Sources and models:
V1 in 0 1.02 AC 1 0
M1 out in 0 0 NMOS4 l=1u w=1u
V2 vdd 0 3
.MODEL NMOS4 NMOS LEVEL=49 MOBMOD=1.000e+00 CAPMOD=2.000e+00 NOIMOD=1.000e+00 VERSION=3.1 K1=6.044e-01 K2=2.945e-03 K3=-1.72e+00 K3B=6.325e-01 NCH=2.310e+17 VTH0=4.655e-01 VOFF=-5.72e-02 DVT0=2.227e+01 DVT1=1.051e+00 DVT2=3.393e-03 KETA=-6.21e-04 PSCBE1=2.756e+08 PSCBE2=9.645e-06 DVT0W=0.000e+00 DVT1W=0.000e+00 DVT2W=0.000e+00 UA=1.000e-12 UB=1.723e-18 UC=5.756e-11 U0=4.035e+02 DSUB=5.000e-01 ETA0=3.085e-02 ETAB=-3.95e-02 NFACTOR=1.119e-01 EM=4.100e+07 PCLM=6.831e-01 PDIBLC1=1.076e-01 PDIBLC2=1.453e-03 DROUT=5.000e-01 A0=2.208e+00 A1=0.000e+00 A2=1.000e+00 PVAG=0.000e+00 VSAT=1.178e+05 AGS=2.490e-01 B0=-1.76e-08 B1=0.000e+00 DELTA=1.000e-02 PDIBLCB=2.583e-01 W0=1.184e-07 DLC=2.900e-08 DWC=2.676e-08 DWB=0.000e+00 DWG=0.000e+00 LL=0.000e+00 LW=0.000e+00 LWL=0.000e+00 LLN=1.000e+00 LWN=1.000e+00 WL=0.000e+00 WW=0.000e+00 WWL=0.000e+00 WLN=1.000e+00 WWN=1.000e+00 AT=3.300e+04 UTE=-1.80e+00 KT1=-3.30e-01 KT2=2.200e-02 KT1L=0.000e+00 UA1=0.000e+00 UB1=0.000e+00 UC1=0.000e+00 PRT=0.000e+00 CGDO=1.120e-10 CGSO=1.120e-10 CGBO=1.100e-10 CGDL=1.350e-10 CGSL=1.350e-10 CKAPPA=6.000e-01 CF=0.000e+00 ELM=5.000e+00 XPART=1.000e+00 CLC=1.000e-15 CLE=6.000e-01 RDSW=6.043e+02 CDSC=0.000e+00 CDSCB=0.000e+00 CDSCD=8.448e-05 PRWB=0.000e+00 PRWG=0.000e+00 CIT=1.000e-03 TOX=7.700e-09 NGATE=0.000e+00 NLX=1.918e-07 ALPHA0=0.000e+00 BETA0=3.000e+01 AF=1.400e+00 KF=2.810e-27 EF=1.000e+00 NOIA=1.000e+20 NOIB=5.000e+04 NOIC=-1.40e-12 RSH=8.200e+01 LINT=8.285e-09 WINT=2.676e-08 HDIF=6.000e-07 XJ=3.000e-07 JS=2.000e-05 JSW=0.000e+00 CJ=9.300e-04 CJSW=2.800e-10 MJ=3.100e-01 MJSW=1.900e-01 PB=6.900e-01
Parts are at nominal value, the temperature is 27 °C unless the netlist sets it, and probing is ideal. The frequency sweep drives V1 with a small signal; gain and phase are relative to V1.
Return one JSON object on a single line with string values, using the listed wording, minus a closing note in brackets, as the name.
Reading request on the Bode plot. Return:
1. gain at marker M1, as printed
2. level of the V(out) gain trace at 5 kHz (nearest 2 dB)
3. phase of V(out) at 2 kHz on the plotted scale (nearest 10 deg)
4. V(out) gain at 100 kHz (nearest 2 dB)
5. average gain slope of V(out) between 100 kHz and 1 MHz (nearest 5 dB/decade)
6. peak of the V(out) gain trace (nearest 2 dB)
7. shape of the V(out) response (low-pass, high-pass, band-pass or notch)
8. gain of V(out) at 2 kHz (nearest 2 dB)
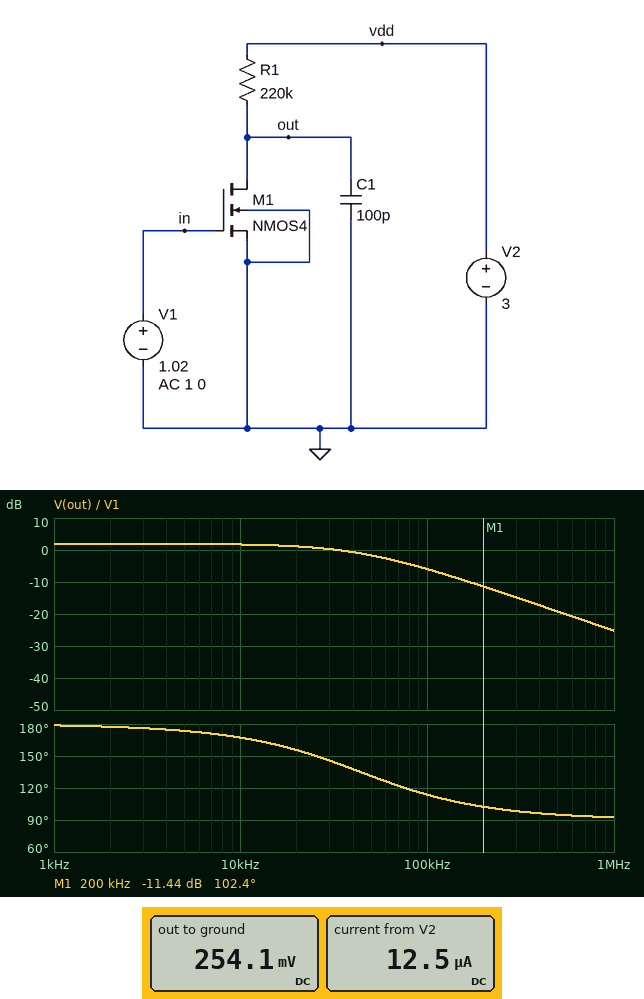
{"gain at marker M1, as printed": "-11.44 dB", "level of the V(out) gain trace at 5 kHz": "2 dB", "phase of V(out) at 2 kHz on the plotted scale": "180 deg", "V(out) gain at 100 kHz": "-6 dB", "average gain slope of V(out) between 100 kHz and 1 MHz": "-20 dB/decade", "peak of the V(out) gain trace": "2 dB", "shape of the V(out) response": "low-pass", "gain of V(out) at 2 kHz": "2 dB"}
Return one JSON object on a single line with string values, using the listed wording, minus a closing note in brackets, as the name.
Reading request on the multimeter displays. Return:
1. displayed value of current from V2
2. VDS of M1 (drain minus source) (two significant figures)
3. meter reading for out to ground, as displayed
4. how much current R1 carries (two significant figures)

{"displayed value of current from V2": "12.5 µA", "VDS of M1 (drain minus source)": "250 mV", "meter reading for out to ground, as displayed": "254.1 mV", "how much current R1 carries": "12 µA"}
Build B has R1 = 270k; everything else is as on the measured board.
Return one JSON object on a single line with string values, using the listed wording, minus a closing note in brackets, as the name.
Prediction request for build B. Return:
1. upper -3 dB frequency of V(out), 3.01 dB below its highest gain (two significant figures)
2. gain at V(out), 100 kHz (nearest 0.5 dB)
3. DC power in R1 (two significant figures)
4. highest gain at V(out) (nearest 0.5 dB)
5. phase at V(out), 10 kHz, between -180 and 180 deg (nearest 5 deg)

{"upper -3 dB frequency of V(out), 3.01 dB below its highest gain": "64 kHz", "gain at V(out), 100 kHz": "-9.5 dB", "DC power in R1": "29 µW", "highest gain at V(out)": "-4.0 dB", "phase at V(out), 10 kHz, between -180 and 180 deg": "170 deg"}
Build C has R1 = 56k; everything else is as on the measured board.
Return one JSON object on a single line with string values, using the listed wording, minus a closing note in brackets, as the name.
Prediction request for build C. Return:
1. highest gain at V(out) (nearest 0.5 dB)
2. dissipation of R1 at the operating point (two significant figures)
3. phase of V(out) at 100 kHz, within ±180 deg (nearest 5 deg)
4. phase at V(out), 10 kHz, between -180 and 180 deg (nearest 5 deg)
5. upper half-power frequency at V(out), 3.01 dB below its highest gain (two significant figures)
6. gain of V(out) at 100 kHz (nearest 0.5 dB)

{"highest gain at V(out)": "9.5 dB", "dissipation of R1 at the operating point": "13 µW", "phase of V(out) at 100 kHz, within ±180 deg": "105 deg", "phase at V(out), 10 kHz, between -180 and 180 deg": "160 deg", "upper half-power frequency at V(out), 3.01 dB below its highest gain": "29 kHz", "gain of V(out) at 100 kHz": "-2.0 dB"}
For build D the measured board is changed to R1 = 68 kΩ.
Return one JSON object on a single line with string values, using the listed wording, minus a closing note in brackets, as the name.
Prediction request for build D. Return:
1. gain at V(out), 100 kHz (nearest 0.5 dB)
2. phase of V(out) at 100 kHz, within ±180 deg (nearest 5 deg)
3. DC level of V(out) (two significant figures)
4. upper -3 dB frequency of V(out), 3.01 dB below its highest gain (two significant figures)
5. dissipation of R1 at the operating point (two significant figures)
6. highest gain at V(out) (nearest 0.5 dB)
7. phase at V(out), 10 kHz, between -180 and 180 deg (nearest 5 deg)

{"gain at V(out), 100 kHz": "-1.5 dB", "phase of V(out) at 100 kHz, within ±180 deg": "105 deg", "DC level of V(out)": "2.0 V", "upper -3 dB frequency of V(out), 3.01 dB below its highest gain": "24 kHz", "dissipation of R1 at the operating point": "15 µW", "highest gain at V(out)": "11.0 dB", "phase at V(out), 10 kHz, between -180 and 180 deg": "155 deg"}
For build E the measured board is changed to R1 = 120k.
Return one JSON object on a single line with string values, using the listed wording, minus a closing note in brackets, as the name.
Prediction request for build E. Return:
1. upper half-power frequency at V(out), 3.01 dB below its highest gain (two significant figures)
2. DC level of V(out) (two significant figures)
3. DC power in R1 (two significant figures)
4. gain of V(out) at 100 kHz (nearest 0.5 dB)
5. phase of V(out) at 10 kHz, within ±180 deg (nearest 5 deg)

{"upper half-power frequency at V(out), 3.01 dB below its highest gain": "14 kHz", "DC level of V(out)": "1.2 V", "DC power in R1": "27 µW", "gain of V(out) at 100 kHz": "-1.5 dB", "phase of V(out) at 10 kHz, within ±180 deg": "145 deg"}
